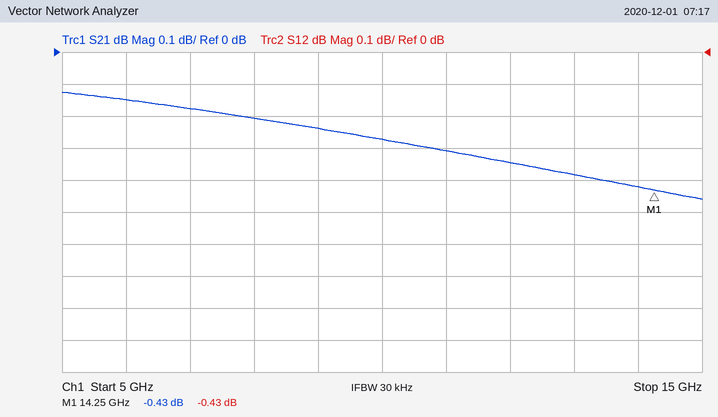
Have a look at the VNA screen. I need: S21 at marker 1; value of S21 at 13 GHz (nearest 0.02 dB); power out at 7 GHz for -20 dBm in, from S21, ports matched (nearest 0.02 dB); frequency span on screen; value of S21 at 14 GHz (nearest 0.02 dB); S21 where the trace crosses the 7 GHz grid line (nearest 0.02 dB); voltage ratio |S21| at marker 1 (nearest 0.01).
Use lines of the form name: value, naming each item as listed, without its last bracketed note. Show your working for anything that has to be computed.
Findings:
S21 at marker 1: -0.43 dB
value of S21 at 13 GHz: -0.38 dB
power out at 7 GHz for -20 dBm in, from S21, ports matched: -20 dBm + (-0.18 dB) = -20.18 dBm
frequency span on screen: 10 GHz
value of S21 at 14 GHz: -0.42 dB
S21 where the trace crosses the 7 GHz grid line: -0.18 dB
voltage ratio |S21| at marker 1: 10^(-0.43/20) ≈ 0.95
